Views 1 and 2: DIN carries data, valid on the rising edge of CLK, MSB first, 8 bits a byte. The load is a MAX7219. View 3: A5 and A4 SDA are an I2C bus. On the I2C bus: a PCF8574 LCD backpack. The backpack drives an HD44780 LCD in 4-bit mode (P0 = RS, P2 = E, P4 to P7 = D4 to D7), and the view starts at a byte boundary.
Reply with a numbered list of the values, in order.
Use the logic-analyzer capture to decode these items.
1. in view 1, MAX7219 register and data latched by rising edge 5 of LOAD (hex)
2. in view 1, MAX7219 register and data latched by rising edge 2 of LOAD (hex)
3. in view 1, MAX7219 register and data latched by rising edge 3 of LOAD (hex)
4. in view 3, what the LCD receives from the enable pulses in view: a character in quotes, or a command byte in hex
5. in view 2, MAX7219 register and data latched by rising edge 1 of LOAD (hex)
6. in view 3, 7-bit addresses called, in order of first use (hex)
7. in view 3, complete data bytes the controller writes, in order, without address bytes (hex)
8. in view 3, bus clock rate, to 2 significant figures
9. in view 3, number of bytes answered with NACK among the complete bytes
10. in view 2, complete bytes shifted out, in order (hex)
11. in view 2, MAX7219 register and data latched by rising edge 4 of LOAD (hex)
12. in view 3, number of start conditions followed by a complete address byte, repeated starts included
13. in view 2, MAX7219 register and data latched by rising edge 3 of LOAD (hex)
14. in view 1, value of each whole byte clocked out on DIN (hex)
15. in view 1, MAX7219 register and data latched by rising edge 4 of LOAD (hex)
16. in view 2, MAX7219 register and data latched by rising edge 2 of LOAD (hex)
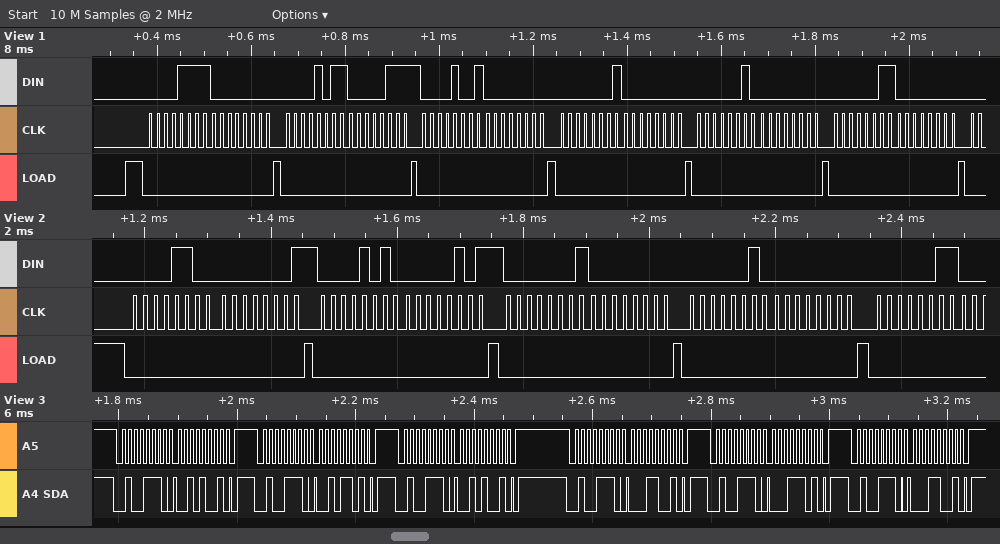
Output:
1. register 0x1, data 0x00
2. register 0xF, data 0x00
3. register 0xB, data 0x07
4. '!'
5. register 0xC, data 0x01
6. 0x27
7. 29 2D 29 19 1D 19
8. 100 kHz
9. 0
10. 0C 01 0A 05 01 00 02 00 03
11. register 0x2, data 0x00
12. 6
13. register 0x1, data 0x00
14. 0F 00 0B 07 09 00 01 00 02 00 03 00
15. register 0x9, data 0x00
16. register 0xA, data 0x05
